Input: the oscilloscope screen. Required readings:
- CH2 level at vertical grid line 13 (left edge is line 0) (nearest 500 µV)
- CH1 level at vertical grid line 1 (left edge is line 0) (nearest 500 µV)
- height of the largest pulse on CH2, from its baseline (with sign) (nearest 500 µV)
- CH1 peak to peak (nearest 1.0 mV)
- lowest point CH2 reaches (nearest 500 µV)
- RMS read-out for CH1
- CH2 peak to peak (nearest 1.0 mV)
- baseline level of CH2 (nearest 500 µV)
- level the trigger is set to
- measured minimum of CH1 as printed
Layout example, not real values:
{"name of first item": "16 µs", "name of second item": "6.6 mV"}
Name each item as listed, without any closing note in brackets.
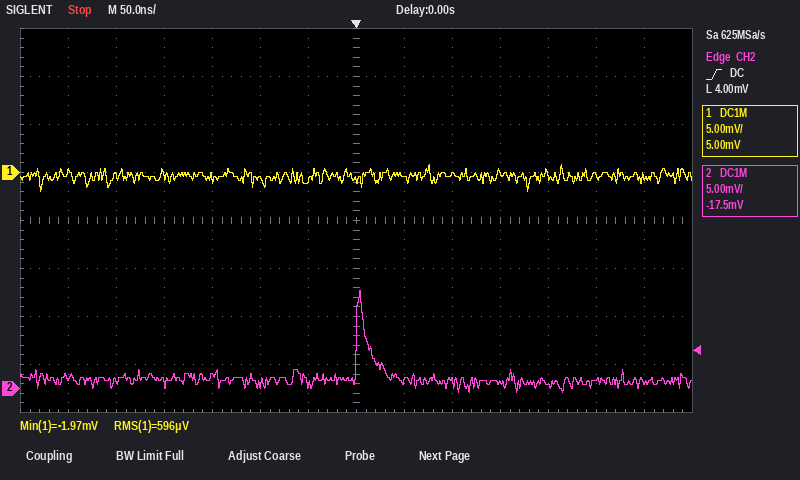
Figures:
{"CH2 level at vertical grid line 13 (left edge is line 0)": "500 µV", "CH1 level at vertical grid line 1 (left edge is line 0)": "0.0 mV", "height of the largest pulse on CH2, from its baseline (with sign)": "+9.5 mV", "CH1 peak to peak": "3.0 mV", "lowest point CH2 reaches": "-500 µV", "RMS read-out for CH1": "596 µV", "CH2 peak to peak": "11.0 mV", "baseline level of CH2": "1.0 mV", "level the trigger is set to": "4.00 mV", "measured minimum of CH1 as printed": "-1.97 mV"}
